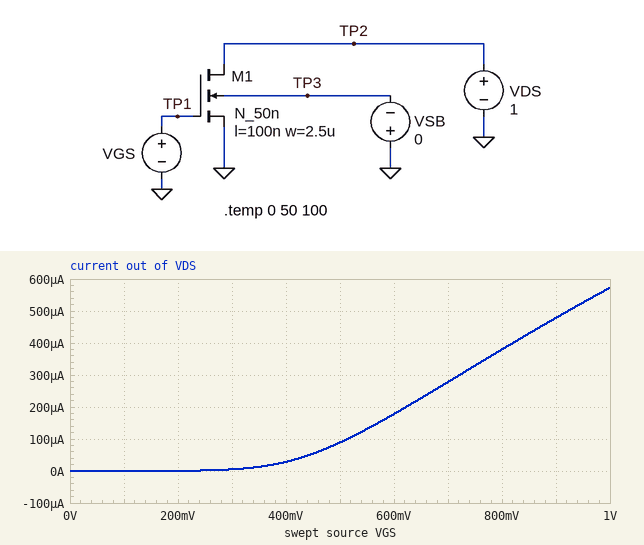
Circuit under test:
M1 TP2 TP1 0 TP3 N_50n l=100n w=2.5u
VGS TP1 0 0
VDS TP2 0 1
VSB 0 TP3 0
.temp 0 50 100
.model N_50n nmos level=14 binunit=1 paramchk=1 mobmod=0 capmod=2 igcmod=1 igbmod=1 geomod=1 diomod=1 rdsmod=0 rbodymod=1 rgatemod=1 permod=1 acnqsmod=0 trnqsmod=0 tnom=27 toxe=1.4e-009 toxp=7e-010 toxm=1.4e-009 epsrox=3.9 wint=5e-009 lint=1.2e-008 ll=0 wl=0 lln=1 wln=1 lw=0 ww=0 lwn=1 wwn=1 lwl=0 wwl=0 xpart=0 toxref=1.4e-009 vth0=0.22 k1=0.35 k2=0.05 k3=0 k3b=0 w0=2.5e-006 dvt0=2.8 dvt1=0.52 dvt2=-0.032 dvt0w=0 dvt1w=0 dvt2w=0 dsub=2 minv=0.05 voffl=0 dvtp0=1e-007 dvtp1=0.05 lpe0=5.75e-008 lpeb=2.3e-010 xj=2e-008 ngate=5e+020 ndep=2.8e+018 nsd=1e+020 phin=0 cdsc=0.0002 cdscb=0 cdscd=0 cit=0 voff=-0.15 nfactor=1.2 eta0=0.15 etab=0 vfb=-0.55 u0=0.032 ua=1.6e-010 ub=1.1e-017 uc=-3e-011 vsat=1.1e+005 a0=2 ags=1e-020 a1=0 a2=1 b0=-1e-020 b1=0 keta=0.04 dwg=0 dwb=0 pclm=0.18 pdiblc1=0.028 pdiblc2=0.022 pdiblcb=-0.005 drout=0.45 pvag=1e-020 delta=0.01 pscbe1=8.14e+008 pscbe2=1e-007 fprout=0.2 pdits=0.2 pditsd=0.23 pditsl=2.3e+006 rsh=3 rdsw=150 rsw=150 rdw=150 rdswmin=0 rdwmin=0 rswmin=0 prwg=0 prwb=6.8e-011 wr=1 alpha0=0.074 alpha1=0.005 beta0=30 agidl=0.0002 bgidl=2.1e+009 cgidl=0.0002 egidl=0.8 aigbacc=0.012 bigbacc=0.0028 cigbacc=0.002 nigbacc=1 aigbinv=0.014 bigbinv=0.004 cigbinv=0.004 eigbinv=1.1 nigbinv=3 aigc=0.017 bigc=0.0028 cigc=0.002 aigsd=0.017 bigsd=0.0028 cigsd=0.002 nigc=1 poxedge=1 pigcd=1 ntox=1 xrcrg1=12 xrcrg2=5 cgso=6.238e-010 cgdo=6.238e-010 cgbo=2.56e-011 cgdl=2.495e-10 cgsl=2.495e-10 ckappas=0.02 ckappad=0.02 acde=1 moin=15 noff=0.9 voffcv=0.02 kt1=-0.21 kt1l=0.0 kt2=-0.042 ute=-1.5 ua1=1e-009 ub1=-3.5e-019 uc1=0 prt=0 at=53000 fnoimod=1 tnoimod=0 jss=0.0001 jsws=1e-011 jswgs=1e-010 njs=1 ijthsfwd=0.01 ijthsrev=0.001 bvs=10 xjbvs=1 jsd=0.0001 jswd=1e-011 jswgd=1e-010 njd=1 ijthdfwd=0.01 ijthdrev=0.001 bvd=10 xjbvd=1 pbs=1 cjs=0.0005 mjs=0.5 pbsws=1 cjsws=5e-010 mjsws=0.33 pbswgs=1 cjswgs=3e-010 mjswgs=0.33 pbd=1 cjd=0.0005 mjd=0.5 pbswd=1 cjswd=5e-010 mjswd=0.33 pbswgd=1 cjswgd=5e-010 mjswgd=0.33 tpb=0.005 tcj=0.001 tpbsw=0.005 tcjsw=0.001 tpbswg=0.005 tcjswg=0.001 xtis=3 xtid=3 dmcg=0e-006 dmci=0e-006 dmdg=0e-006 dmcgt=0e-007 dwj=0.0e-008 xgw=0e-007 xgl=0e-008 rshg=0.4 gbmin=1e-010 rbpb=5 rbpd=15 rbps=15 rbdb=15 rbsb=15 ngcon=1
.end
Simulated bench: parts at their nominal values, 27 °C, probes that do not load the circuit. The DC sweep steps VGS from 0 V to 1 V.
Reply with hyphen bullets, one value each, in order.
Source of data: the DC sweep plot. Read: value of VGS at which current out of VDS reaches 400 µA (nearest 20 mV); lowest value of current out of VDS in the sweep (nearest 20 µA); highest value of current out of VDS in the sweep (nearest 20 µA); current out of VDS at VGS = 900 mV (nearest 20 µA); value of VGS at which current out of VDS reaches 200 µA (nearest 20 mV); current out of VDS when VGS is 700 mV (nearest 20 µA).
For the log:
- 820 mV
- 0 A
- 580 µA
- 480 µA
- 620 mV
- 280 µA
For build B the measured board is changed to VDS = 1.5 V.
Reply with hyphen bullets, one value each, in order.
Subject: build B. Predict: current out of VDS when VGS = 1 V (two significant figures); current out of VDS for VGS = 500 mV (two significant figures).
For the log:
- 620 µA
- 100 µA
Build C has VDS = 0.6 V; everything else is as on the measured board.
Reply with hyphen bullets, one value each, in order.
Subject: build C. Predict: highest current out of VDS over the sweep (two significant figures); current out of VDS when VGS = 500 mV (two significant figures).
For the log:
- 530 µA
- 79 µA
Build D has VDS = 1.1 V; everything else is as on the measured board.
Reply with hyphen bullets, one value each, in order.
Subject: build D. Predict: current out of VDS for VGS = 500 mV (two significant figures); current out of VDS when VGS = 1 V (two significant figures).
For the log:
- 92 µA
- 580 µA
